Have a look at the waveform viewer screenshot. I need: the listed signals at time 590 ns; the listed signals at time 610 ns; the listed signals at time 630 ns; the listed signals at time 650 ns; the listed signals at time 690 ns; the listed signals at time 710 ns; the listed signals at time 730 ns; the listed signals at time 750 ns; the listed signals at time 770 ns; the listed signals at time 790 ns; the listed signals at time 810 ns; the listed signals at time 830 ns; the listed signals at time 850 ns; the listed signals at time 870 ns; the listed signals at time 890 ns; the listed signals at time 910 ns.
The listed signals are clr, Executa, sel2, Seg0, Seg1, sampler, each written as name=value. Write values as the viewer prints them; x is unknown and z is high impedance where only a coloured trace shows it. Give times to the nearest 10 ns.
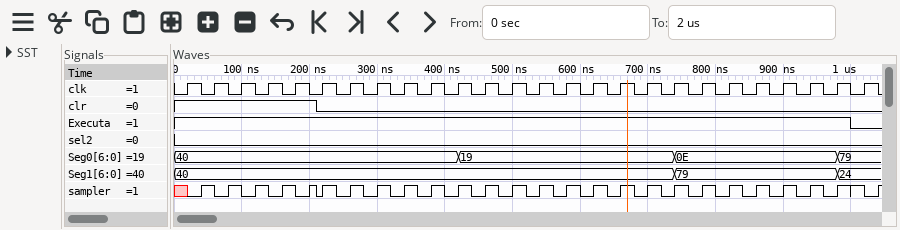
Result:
clr=0, Executa=1, sel2=0, Seg0=19, Seg1=40, sampler=1
clr=0, Executa=1, sel2=0, Seg0=19, Seg1=40, sampler=0
clr=0, Executa=1, sel2=0, Seg0=19, Seg1=40, sampler=1
clr=0, Executa=1, sel2=0, Seg0=19, Seg1=40, sampler=0
clr=0, Executa=1, sel2=0, Seg0=19, Seg1=40, sampler=0
clr=0, Executa=1, sel2=0, Seg0=19, Seg1=40, sampler=1
clr=0, Executa=1, sel2=0, Seg0=19, Seg1=40, sampler=0
clr=0, Executa=1, sel2=0, Seg0=0E, Seg1=79, sampler=1
clr=0, Executa=1, sel2=0, Seg0=0E, Seg1=79, sampler=0
clr=0, Executa=1, sel2=0, Seg0=0E, Seg1=79, sampler=1
clr=0, Executa=1, sel2=0, Seg0=0E, Seg1=79, sampler=0
clr=0, Executa=1, sel2=0, Seg0=0E, Seg1=79, sampler=1
clr=0, Executa=1, sel2=0, Seg0=0E, Seg1=79, sampler=0
clr=0, Executa=1, sel2=0, Seg0=0E, Seg1=79, sampler=1
clr=0, Executa=1, sel2=0, Seg0=0E, Seg1=79, sampler=0
clr=0, Executa=1, sel2=0, Seg0=0E, Seg1=79, sampler=1
